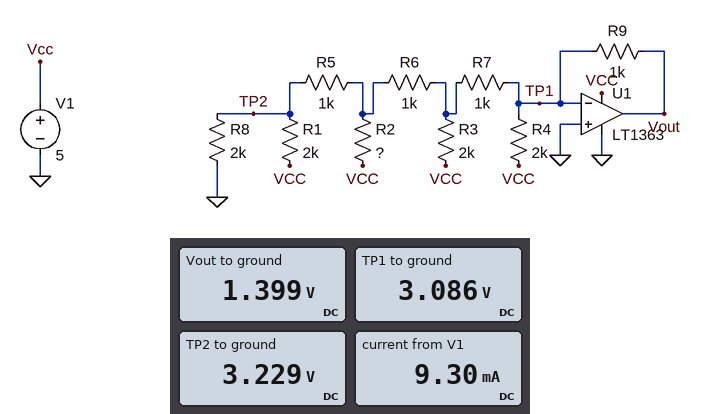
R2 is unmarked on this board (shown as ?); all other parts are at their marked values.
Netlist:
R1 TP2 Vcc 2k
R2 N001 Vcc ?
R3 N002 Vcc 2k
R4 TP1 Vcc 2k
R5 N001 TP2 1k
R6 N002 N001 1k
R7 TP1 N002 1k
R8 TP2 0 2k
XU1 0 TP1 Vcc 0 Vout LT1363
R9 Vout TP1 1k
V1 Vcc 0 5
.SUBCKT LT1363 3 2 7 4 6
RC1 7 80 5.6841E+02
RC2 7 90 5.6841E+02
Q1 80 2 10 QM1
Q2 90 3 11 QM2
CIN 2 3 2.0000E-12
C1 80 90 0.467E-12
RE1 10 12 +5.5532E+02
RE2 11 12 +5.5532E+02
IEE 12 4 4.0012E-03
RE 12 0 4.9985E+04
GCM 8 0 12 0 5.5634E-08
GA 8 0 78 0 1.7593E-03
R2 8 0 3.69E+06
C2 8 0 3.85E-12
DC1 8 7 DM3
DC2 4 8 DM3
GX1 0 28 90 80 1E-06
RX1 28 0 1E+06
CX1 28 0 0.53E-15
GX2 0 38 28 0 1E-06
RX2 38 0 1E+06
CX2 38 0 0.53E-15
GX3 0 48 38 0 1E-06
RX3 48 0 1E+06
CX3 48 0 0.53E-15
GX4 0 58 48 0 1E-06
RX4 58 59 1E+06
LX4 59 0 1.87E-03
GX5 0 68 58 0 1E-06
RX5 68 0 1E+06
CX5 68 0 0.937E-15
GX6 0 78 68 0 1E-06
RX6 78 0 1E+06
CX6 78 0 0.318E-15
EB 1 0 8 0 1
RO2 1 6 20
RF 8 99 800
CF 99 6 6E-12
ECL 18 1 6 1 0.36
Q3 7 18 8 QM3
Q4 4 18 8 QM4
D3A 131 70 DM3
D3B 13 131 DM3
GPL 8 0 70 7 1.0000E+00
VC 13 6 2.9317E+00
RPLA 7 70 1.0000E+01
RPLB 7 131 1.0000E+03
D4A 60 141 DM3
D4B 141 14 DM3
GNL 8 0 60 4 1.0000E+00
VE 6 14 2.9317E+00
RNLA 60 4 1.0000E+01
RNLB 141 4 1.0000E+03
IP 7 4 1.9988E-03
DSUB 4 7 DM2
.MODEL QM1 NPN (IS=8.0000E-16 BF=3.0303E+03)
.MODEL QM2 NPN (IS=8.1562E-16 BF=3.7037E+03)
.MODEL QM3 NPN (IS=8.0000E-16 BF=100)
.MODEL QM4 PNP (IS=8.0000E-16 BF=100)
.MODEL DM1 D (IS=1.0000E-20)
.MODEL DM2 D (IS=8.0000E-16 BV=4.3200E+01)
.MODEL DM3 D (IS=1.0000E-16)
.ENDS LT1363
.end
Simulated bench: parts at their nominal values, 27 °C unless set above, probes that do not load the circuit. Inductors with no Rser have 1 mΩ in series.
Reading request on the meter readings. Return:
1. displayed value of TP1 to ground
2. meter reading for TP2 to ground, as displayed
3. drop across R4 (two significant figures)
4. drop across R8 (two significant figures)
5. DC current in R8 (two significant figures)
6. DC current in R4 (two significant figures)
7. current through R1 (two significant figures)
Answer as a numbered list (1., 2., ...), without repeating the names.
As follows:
1. 3.086 V
2. 3.229 V
3. 1.9 V
4. 3.2 V
5. 1.6 mA
6. 960 µA
7. 890 µA
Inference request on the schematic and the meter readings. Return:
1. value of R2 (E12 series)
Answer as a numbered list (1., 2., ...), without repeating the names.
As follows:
1. 1.2 kΩ
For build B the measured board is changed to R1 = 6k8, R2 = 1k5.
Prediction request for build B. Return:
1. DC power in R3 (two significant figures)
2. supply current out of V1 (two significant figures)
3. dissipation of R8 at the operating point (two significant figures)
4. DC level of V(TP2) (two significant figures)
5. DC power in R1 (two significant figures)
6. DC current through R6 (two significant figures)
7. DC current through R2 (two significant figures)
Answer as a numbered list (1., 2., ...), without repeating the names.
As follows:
1. 910 µW
2. 8.9 mA
3. 3.5 mW
4. 2.6 V
5. 820 µW
6. 43 µA
7. 930 µA
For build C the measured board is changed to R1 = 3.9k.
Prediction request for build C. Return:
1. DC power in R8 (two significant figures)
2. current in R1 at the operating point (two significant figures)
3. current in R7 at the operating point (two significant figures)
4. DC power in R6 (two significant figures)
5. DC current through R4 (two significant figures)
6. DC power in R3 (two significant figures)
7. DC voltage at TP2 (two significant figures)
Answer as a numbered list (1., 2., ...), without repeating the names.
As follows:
1. 4.2 mW
2. 540 µA
3. 690 µA
4. 4.6 µW
5. 970 µA
6. 780 µW
7. 2.9 V
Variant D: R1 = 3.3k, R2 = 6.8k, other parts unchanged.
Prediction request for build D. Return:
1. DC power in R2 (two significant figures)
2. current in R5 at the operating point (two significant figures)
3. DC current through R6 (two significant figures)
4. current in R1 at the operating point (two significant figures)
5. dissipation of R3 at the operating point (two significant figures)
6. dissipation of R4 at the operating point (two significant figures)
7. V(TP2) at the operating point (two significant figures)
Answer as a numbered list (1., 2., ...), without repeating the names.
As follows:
1. 510 µW
2. 560 µA
3. 290 µA
4. 730 µA
5. 1.2 mW
6. 2.1 mW
7. 2.6 V
